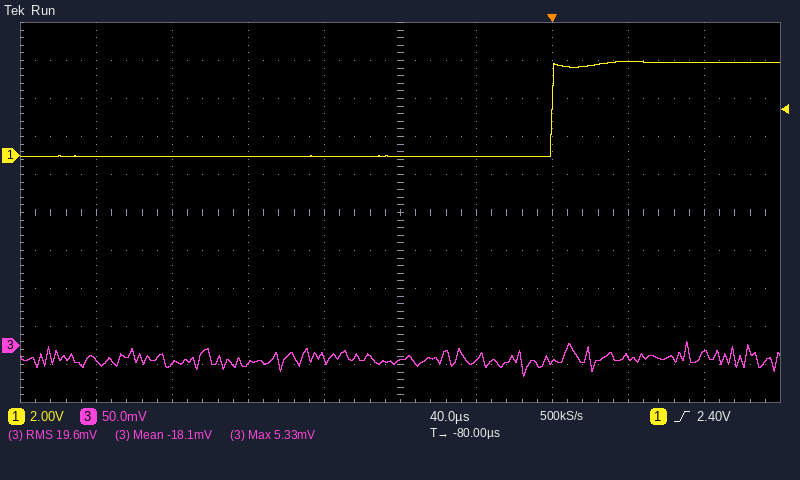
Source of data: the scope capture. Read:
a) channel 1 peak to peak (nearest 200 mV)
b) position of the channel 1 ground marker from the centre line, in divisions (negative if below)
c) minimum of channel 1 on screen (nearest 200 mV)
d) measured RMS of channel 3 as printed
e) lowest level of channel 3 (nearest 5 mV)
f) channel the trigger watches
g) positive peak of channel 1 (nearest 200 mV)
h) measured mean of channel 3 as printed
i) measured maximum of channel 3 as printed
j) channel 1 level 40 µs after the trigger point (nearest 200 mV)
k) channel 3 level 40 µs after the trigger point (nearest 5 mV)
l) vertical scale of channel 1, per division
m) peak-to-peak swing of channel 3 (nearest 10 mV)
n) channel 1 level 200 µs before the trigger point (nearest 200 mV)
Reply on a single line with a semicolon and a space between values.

5.0 V; +1.5 div; 0.0 V; 19.6 mV; -40 mV; channel 1; 5.0 V; -18.1 mV; 5.33 mV; 5.0 V; -15 mV; 2 V; 50 mV; 0.0 V
